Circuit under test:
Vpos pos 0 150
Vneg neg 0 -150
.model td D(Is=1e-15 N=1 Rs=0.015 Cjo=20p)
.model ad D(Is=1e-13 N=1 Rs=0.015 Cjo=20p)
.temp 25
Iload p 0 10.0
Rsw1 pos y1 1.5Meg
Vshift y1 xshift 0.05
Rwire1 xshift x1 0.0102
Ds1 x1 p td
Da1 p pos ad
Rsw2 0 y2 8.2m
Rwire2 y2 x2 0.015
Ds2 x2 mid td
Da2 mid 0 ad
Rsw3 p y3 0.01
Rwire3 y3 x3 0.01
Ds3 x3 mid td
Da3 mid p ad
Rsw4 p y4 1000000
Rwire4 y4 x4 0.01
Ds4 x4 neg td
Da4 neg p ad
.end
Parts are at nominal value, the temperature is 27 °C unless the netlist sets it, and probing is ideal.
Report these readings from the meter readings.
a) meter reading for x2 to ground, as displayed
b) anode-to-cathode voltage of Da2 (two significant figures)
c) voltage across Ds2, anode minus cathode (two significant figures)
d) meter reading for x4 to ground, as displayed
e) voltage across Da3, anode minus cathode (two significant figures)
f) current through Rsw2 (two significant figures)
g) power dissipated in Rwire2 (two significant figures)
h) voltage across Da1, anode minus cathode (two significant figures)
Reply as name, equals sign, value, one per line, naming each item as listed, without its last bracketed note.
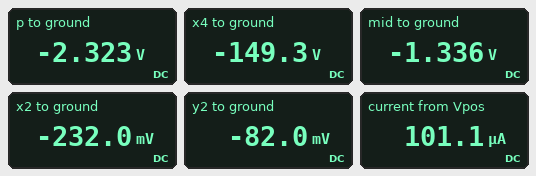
meter reading for x2 to ground, as displayed = -232.0 mV
anode-to-cathode voltage of Da2 = -1.3 V
voltage across Ds2, anode minus cathode = 1.1 V
meter reading for x4 to ground, as displayed = -149.3 V
voltage across Da3, anode minus cathode = 990 mV
current through Rsw2 = 10 A
power dissipated in Rwire2 = 1.5 W
voltage across Da1, anode minus cathode = -150 V
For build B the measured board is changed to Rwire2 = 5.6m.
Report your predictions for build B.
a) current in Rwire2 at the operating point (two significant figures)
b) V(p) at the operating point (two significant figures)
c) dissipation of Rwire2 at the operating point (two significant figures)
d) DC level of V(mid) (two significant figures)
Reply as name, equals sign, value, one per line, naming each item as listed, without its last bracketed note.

current in Rwire2 at the operating point = 10 A
V(p) at the operating point = -2.2 V
dissipation of Rwire2 at the operating point = 560 mW
DC level of V(mid) = -1.2 V
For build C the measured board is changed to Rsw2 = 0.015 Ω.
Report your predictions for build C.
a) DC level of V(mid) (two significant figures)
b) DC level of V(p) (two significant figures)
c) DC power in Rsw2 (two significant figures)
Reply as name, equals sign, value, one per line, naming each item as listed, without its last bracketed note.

DC level of V(mid) = -1.4 V
DC level of V(p) = -2.4 V
DC power in Rsw2 = 1.5 W
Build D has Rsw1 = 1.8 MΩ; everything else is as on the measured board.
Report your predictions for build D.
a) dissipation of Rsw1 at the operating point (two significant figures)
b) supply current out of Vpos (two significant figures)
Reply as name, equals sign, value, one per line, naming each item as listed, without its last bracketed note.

dissipation of Rsw1 at the operating point = 13 mW
supply current out of Vpos = 84 µA
